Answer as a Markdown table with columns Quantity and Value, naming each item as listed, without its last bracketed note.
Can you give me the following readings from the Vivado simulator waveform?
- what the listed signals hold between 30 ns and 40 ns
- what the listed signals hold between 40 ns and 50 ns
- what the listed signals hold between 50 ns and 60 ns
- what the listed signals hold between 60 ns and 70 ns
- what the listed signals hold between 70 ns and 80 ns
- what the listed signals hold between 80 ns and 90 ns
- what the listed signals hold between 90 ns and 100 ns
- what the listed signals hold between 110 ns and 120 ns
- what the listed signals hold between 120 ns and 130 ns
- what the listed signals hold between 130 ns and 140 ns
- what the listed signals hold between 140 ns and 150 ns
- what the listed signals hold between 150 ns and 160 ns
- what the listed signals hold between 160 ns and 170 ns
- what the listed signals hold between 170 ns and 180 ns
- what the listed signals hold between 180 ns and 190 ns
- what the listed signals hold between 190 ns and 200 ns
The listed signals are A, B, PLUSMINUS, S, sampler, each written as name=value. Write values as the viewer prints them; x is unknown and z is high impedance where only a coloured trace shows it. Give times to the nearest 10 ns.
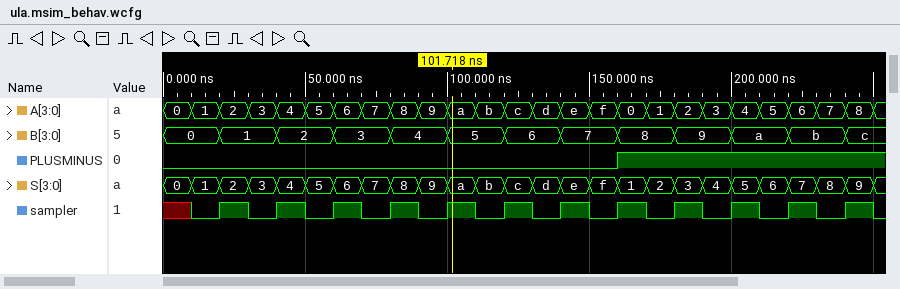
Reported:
| Quantity | Value |
|---|---|
| what the listed signals hold between 30 ns and 40 ns | A=3, B=1, PLUSMINUS=0, S=3, sampler=0 |
| what the listed signals hold between 40 ns and 50 ns | A=4, B=2, PLUSMINUS=0, S=4, sampler=1 |
| what the listed signals hold between 50 ns and 60 ns | A=5, B=2, PLUSMINUS=0, S=5, sampler=0 |
| what the listed signals hold between 60 ns and 70 ns | A=6, B=3, PLUSMINUS=0, S=6, sampler=1 |
| what the listed signals hold between 70 ns and 80 ns | A=7, B=3, PLUSMINUS=0, S=7, sampler=0 |
| what the listed signals hold between 80 ns and 90 ns | A=8, B=4, PLUSMINUS=0, S=8, sampler=1 |
| what the listed signals hold between 90 ns and 100 ns | A=9, B=4, PLUSMINUS=0, S=9, sampler=0 |
| what the listed signals hold between 110 ns and 120 ns | A=b, B=5, PLUSMINUS=0, S=b, sampler=0 |
| what the listed signals hold between 120 ns and 130 ns | A=c, B=6, PLUSMINUS=0, S=c, sampler=1 |
| what the listed signals hold between 130 ns and 140 ns | A=d, B=6, PLUSMINUS=0, S=d, sampler=0 |
| what the listed signals hold between 140 ns and 150 ns | A=e, B=7, PLUSMINUS=0, S=e, sampler=1 |
| what the listed signals hold between 150 ns and 160 ns | A=f, B=7, PLUSMINUS=0, S=f, sampler=0 |
| what the listed signals hold between 160 ns and 170 ns | A=0, B=8, PLUSMINUS=1, S=1, sampler=1 |
| what the listed signals hold between 170 ns and 180 ns | A=1, B=8, PLUSMINUS=1, S=2, sampler=0 |
| what the listed signals hold between 180 ns and 190 ns | A=2, B=9, PLUSMINUS=1, S=3, sampler=1 |
| what the listed signals hold between 190 ns and 200 ns | A=3, B=9, PLUSMINUS=1, S=4, sampler=0 |
